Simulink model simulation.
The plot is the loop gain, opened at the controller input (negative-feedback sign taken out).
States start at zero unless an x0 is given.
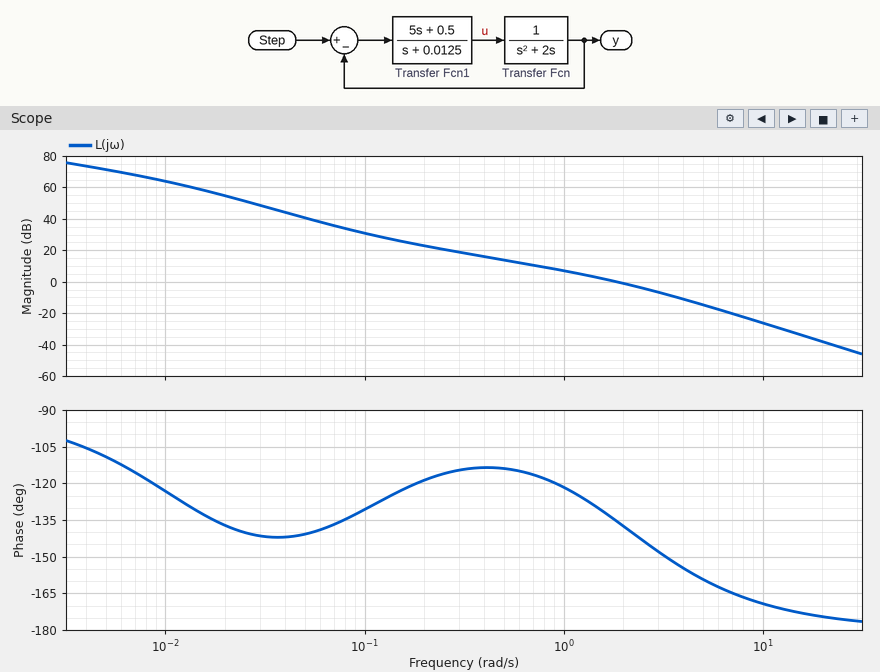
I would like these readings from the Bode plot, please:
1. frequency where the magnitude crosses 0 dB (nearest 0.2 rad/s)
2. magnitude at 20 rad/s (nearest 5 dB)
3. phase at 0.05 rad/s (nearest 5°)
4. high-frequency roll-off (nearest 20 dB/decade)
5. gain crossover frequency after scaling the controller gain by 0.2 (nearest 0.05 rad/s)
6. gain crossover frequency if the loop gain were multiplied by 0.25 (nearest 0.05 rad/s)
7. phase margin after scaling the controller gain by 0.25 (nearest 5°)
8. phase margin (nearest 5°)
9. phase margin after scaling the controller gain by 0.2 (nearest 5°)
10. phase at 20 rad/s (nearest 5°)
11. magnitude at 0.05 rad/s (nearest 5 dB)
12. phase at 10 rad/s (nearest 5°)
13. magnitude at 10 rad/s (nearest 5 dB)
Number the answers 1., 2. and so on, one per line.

1. 1.8 rad/s
2. -40 dB
3. -140°
4. -40 dB/decade
5. 0.50 rad/s
6. 0.60 rad/s
7. 65°
8. 45°
9. 65°
10. -175°
11. 40 dB
12. -170°
13. -25 dB
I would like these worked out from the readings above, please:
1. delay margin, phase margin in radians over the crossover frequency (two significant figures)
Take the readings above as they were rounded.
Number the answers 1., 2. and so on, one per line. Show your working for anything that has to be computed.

1. 45 × π / 180 / 1.8 = 0.44 s
